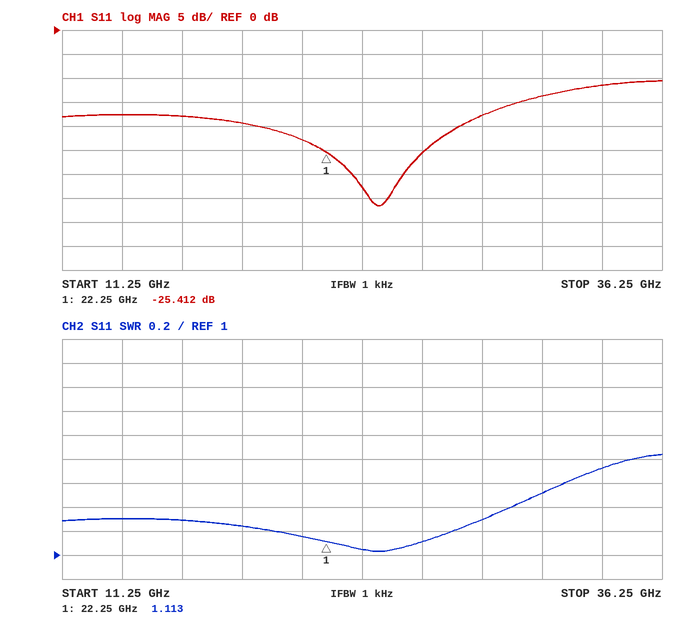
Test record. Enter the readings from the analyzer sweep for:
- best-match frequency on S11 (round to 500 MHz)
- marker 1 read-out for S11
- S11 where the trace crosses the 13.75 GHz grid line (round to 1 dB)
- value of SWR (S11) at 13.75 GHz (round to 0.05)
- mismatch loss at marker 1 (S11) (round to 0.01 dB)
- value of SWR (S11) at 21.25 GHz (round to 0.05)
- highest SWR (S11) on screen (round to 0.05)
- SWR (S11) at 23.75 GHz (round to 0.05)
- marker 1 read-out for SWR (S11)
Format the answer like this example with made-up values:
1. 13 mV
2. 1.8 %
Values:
1. 24.5 GHz
2. -25.412 dB
3. -18 dB
4. 1.30
5. 0.01 dB
6. 1.15
7. 1.85
8. 1.05
9. 1.113
